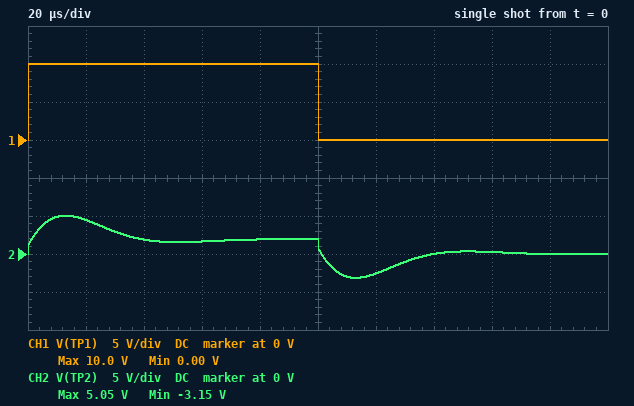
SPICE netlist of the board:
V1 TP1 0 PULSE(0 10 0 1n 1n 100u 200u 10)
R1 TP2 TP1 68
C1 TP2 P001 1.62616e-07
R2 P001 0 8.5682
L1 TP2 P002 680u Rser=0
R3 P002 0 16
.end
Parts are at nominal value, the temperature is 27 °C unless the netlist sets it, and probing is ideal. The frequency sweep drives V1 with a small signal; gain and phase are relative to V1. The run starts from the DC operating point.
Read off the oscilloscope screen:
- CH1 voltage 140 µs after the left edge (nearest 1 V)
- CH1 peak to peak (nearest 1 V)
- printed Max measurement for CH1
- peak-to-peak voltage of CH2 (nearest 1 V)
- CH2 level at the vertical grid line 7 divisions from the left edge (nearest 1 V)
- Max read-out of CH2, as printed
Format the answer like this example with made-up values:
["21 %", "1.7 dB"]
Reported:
["0 V", "10 V", "10.0 V", "8 V", "0 V", "5.05 V"]
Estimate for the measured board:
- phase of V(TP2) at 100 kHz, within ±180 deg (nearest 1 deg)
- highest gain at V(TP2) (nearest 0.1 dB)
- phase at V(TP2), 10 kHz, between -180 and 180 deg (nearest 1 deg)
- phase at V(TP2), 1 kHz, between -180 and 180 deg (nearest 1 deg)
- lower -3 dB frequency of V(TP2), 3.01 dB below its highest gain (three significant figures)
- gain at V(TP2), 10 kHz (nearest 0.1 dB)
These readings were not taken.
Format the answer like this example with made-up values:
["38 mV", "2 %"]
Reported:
["-40 deg", "-2.8 dB", "24 deg", "11 deg", "8.70 kHz", "-4.8 dB"]
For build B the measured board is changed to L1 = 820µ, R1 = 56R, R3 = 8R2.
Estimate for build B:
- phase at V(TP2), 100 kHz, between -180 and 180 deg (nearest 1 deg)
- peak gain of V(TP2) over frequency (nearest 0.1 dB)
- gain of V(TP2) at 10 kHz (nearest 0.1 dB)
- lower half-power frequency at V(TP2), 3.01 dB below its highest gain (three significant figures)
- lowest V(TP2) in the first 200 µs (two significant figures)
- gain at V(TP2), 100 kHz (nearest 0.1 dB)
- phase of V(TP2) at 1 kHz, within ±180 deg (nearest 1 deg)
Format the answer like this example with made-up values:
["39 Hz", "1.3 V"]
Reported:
["-39 deg", "-1.5 dB", "-2.4 dB", "7.29 kHz", "-4.5 V", "-13.9 dB", "27 deg"]
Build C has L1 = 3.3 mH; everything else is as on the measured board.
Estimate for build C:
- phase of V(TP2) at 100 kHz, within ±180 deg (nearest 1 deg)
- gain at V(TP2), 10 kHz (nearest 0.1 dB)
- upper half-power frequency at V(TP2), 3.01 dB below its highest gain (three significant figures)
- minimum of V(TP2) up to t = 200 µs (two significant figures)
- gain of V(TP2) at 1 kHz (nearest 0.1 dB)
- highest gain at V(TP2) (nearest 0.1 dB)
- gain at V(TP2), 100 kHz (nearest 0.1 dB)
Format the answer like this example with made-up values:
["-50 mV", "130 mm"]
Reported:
["-41 deg", "-1.2 dB", "17.1 kHz", "-5.1 V", "-10.3 dB", "-0.7 dB", "-15.4 dB"]
